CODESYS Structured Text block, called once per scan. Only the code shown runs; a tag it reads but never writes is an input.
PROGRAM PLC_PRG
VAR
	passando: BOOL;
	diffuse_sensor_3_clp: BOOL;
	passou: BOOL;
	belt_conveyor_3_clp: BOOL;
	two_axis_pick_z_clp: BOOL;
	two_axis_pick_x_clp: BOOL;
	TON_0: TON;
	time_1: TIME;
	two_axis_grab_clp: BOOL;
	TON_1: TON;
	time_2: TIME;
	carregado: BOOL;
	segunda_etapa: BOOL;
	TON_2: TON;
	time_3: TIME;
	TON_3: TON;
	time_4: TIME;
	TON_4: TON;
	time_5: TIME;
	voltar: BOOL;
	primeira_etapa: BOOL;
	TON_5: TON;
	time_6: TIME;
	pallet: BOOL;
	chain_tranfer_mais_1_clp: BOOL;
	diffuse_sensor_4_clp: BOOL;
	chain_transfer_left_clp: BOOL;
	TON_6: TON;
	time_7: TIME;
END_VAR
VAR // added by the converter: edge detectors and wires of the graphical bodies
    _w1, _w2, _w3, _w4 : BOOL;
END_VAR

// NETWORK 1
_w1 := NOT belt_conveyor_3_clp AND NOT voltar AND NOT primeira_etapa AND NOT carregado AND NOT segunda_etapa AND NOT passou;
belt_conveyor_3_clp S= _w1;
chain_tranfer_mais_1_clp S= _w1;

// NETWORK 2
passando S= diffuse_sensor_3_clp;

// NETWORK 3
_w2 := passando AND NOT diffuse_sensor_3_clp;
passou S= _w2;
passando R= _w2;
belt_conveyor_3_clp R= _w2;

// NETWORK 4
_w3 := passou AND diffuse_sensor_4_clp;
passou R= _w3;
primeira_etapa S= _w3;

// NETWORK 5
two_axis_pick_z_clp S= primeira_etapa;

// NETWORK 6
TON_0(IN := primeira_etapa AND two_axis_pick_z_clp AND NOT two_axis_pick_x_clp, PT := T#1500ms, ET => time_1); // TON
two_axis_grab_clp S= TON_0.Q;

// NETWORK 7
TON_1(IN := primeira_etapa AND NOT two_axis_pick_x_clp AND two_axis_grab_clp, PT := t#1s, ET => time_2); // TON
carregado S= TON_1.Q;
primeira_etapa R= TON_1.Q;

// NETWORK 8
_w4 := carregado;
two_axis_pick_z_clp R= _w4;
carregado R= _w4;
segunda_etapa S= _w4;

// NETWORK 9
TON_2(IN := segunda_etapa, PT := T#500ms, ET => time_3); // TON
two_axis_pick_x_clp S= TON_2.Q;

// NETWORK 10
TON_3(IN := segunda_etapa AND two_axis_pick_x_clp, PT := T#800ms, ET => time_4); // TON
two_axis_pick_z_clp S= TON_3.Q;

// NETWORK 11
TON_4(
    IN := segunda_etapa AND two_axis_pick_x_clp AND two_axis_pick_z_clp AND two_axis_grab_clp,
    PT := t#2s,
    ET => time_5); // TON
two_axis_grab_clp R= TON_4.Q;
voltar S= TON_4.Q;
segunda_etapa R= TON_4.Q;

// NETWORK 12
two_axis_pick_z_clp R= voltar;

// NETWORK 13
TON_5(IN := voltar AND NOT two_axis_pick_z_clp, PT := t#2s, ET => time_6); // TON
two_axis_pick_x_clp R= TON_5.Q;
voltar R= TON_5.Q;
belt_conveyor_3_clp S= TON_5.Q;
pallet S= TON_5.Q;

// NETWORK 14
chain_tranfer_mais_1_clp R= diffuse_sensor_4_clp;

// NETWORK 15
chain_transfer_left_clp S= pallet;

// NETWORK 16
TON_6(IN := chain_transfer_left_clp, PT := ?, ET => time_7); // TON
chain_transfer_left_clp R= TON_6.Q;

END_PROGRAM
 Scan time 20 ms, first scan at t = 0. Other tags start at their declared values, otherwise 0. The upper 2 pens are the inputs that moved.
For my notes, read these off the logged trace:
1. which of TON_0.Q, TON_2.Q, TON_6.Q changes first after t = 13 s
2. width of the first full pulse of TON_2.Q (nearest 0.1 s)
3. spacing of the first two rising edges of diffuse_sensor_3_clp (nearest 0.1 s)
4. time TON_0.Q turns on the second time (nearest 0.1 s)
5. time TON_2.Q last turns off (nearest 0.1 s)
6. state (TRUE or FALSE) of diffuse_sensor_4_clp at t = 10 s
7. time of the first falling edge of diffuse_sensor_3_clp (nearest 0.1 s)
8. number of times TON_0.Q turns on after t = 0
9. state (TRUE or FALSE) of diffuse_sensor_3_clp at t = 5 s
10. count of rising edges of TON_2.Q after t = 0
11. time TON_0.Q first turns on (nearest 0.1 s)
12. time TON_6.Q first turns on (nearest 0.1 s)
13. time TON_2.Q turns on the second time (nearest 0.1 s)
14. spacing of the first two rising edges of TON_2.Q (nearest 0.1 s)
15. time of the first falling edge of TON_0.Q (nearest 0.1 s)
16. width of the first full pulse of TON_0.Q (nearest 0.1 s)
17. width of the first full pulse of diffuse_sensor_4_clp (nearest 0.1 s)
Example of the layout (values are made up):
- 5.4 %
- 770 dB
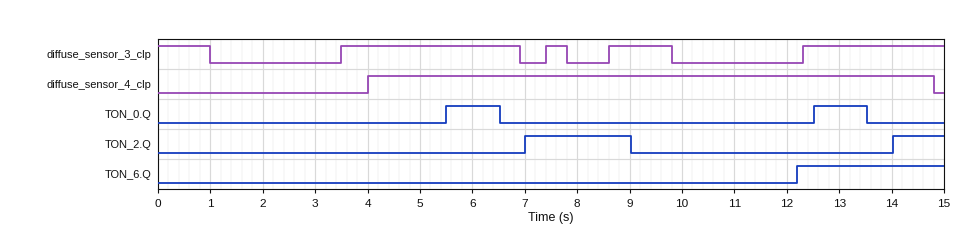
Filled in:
- TON_0.Q
- 2.0 s
- 3.9 s
- 12.5 s
- 9.0 s
- TRUE
- 1.0 s
- 2
- TRUE
- 2
- 5.5 s
- 12.2 s
- 14.0 s
- 7.0 s
- 6.5 s
- 1.0 s
- 10.8 s
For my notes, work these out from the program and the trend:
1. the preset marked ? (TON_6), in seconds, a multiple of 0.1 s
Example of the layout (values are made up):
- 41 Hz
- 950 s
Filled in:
- 1.2 s
